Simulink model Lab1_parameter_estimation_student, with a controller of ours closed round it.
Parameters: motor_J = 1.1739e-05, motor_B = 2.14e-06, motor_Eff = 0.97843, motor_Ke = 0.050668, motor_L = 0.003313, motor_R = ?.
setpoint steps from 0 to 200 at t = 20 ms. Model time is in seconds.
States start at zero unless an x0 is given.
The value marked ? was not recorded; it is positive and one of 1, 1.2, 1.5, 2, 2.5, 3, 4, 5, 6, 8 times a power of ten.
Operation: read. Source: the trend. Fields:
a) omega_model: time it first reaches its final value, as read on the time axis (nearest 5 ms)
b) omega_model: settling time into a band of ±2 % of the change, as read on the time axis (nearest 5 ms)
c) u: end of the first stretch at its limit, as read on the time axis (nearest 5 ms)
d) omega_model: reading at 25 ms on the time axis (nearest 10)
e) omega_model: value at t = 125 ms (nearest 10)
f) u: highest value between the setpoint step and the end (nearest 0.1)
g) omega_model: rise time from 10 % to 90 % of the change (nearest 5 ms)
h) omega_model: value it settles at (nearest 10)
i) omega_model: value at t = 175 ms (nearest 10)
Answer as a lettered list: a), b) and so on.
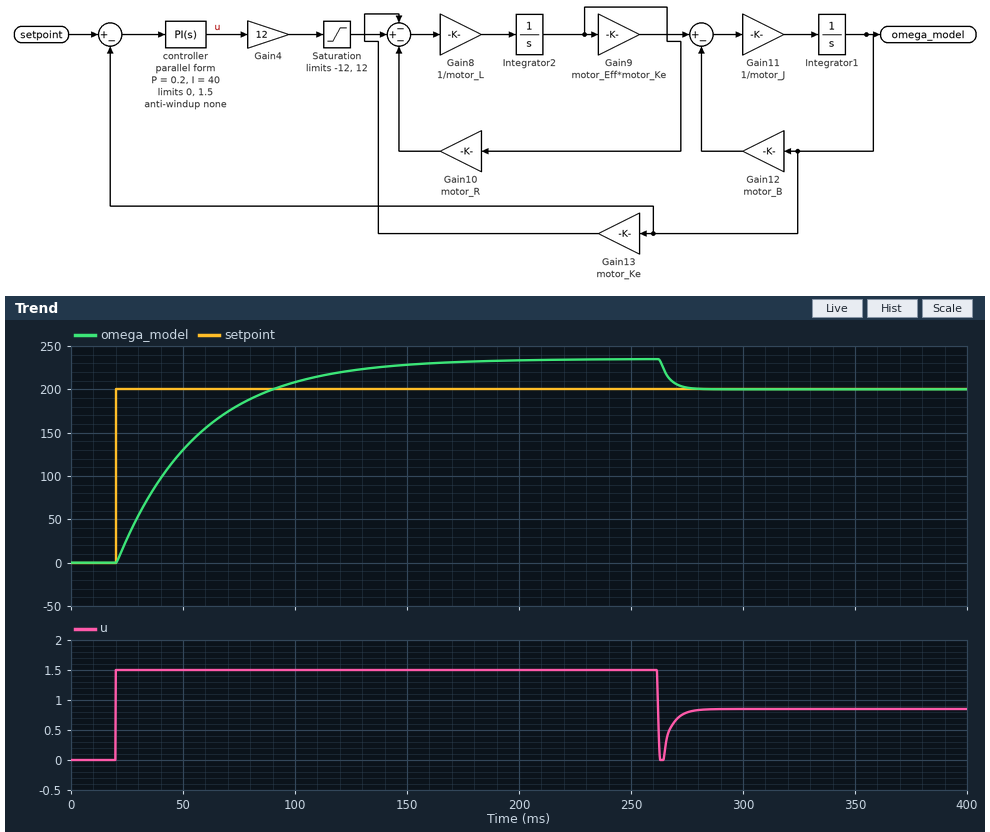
a) 90 ms
b) 270 ms
c) 260 ms
d) 30
e) 220
f) 1.5
g) 50 ms
h) 200
i) 230
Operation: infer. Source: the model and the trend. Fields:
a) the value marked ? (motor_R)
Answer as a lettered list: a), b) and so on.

a) 8
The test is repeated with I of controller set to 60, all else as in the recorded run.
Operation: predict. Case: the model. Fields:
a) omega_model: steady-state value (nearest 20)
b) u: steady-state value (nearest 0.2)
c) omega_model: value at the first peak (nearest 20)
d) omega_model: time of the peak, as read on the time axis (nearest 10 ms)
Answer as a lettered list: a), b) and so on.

a) 200
b) 0.8
c) 240
d) 260 ms
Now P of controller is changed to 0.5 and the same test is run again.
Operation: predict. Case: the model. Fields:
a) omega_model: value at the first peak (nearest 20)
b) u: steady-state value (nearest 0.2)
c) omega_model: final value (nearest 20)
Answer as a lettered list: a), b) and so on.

a) 240
b) 0.8
c) 200
